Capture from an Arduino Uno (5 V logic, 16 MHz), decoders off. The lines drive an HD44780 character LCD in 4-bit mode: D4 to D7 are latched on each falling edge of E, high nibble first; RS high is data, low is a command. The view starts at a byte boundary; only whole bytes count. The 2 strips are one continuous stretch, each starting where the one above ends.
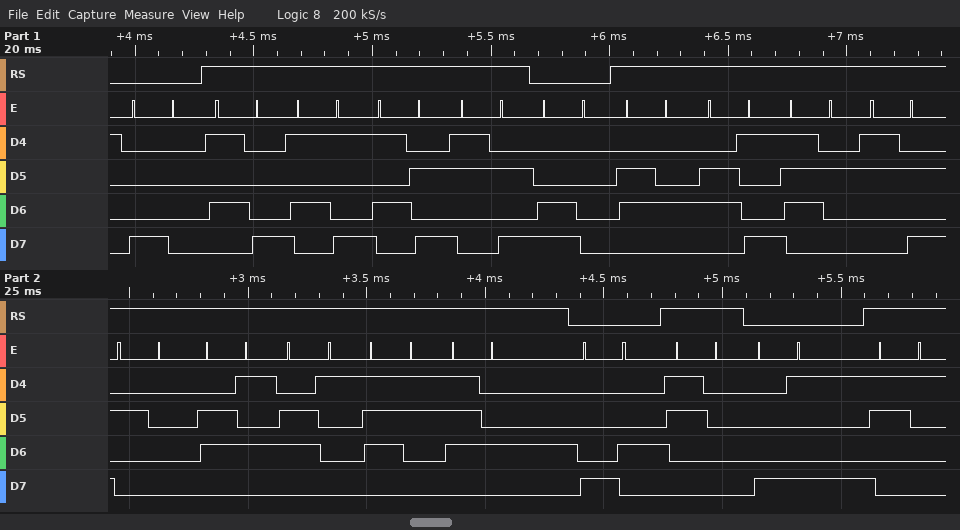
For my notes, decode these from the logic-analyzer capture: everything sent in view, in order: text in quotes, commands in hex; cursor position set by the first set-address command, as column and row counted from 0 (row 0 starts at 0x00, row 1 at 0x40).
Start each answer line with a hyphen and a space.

- 0x80 "XYZ:" 0xC0 "dir: east" 0x84 "0" 0x89 "1"
- column 0, row 0
